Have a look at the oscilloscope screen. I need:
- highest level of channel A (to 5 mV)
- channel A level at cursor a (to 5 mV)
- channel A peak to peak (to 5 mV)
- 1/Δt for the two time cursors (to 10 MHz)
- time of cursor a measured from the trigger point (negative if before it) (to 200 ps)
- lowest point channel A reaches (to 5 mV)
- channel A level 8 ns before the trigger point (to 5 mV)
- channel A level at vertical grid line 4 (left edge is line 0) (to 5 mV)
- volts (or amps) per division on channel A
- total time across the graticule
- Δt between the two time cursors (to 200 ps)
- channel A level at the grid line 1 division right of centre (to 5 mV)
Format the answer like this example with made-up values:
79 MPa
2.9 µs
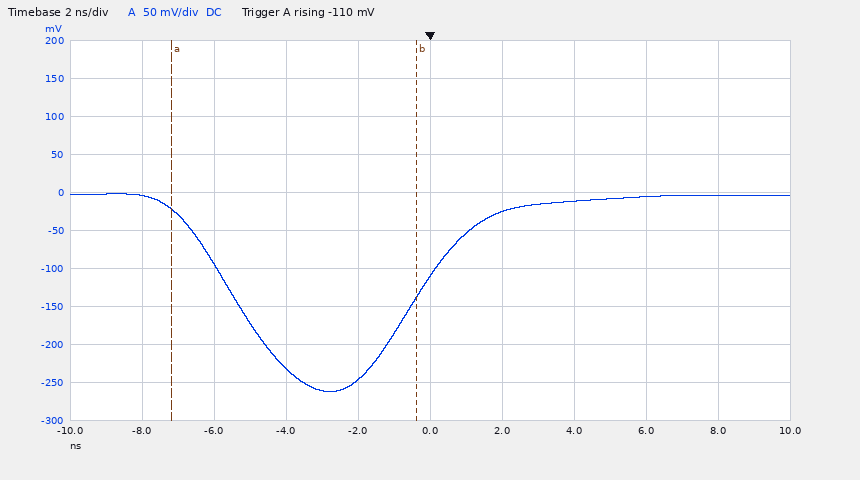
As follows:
0 mV
-20 mV
260 mV
150 MHz
-7.2 ns
-260 mV
-5 mV
-245 mV
50 mV
20 ns
6.8 ns
-25 mV
